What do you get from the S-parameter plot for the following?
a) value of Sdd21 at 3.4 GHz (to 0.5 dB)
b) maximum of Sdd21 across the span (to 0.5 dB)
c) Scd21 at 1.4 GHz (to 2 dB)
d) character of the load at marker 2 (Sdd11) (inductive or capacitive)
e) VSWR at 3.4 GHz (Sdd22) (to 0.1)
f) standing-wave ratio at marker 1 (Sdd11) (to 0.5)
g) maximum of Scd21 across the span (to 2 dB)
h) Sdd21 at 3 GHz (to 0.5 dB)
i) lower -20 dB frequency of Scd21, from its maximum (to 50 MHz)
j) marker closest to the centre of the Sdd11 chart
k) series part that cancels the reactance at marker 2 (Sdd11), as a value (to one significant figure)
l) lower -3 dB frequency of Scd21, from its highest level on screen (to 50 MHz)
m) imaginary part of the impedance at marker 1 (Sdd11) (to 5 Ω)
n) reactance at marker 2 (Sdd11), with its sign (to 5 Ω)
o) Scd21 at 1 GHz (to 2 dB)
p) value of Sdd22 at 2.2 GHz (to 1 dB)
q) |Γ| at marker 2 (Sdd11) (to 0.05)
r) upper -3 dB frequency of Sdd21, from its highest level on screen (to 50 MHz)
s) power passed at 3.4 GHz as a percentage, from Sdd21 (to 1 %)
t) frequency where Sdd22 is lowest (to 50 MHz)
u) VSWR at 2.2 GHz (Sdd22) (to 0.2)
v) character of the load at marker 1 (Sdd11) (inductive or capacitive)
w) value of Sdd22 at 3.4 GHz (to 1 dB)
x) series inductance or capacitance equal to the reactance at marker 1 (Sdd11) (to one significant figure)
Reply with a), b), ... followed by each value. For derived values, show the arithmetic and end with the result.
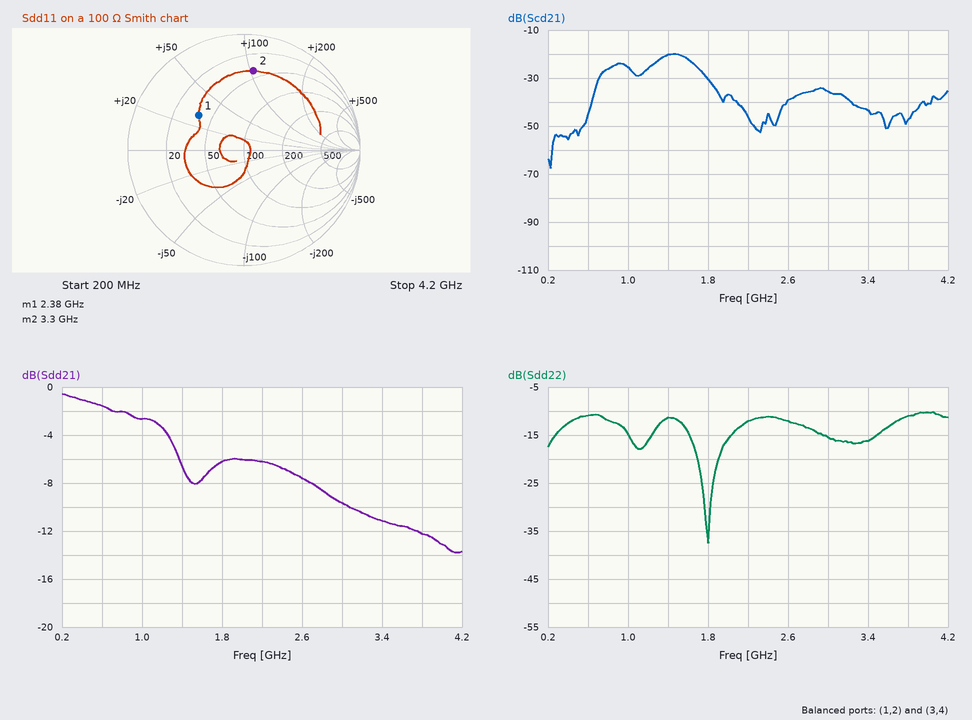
a) -11.0 dB
b) -0.5 dB
c) -20 dB
d) inductive
e) |Γ| = 10^(-16/20) = 0.1585; VSWR = (1 + 0.1585)/(1 − 0.1585) ≈ 1.4
f) 3.0
g) -20 dB
h) -9.5 dB
i) 650 MHz
j) marker 1
k) C = 1/(2π × 3.3 GHz × 105 Ω) ≈ 459 fF, so 500 fF to one significant figure
l) 1.30 GHz
m) +30 Ω
n) +105 Ω
o) -26 dB
p) -12 dB
q) 0.70
r) 1.20 GHz
s) 10^(-11/10) ≈ 8 %
t) 1.80 GHz
u) |Γ| = 10^(-12/20) = 0.2512; VSWR = (1 + 0.2512)/(1 − 0.2512) ≈ 1.67, so 1.6 to the nearest 0.2
v) inductive
w) -16 dB
x) L = 30 Ω/(2π × 2.38 GHz) ≈ 2 nH
